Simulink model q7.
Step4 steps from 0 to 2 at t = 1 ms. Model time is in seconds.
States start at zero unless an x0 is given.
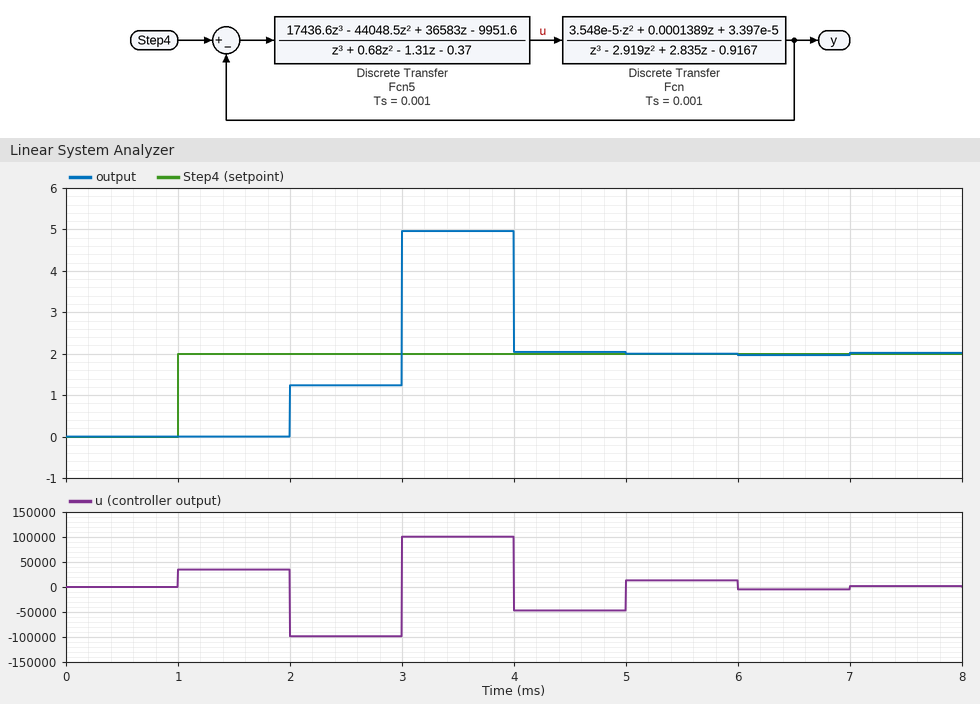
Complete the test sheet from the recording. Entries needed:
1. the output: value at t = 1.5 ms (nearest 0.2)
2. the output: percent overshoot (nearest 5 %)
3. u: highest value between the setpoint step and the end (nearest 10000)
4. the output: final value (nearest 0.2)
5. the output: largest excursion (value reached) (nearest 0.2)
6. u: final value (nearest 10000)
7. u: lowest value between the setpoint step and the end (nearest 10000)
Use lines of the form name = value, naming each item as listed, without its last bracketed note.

the output: value at t = 1.5 ms = 0.0
the output: percent overshoot = 145 %
u: highest value between the setpoint step and the end = 100000
the output: final value = 2.0
the output: largest excursion (value reached) = 5.0
u: final value = 0
u: lowest value between the setpoint step and the end = -100000
